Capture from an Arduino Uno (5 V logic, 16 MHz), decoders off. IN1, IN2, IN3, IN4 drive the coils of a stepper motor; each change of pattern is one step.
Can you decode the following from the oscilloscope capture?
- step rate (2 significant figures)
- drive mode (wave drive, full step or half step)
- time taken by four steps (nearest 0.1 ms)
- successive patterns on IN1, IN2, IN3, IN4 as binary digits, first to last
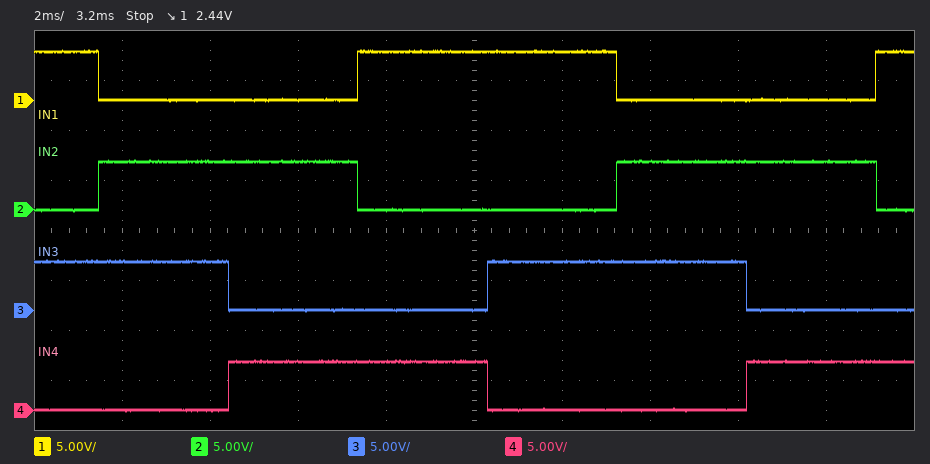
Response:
340 steps/s
full step
11.8 ms
1010 0110 0101 1001 1010 0110 0101 1001
